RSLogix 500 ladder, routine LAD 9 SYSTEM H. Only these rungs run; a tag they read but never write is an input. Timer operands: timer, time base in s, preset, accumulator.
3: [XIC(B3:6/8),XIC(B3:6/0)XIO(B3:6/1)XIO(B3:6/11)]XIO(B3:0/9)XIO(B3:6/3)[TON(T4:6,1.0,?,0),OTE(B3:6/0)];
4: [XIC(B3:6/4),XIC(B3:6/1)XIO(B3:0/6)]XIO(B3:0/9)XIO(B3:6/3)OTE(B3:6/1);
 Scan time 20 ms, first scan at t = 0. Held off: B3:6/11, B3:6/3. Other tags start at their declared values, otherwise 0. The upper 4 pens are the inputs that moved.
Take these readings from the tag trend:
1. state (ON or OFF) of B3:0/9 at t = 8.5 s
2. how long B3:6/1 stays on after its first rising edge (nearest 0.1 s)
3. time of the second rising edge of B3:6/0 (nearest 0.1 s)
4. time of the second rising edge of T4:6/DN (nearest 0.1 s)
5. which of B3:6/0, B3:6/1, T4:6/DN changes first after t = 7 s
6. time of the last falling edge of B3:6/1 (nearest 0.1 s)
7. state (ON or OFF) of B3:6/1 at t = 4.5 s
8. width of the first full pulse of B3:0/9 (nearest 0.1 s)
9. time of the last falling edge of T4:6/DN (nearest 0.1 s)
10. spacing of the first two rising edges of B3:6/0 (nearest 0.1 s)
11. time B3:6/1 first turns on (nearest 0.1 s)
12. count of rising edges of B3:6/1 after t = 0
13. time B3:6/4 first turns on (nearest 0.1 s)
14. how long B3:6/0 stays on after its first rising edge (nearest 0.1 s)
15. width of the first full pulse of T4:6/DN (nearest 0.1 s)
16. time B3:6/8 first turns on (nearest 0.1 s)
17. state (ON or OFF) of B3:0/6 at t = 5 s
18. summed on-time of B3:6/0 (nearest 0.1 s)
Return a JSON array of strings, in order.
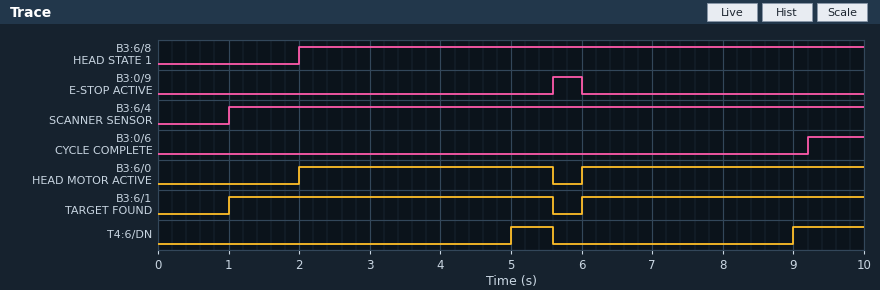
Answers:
["OFF", "4.6 s", "6.0 s", "9.0 s", "T4:6/DN", "5.6 s", "ON", "0.4 s", "5.6 s", "4.0 s", "1.0 s", "2", "1.0 s", "3.6 s", "0.6 s", "2.0 s", "OFF", "7.6 s"]
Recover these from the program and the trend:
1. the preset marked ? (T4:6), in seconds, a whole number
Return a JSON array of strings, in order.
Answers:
["3 s"]
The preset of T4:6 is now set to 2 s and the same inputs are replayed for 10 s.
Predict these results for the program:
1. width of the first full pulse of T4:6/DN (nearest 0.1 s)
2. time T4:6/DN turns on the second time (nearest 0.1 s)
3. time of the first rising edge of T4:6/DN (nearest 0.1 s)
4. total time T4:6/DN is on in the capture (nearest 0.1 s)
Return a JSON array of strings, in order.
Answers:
["1.6 s", "8.0 s", "4.0 s", "3.6 s"]
